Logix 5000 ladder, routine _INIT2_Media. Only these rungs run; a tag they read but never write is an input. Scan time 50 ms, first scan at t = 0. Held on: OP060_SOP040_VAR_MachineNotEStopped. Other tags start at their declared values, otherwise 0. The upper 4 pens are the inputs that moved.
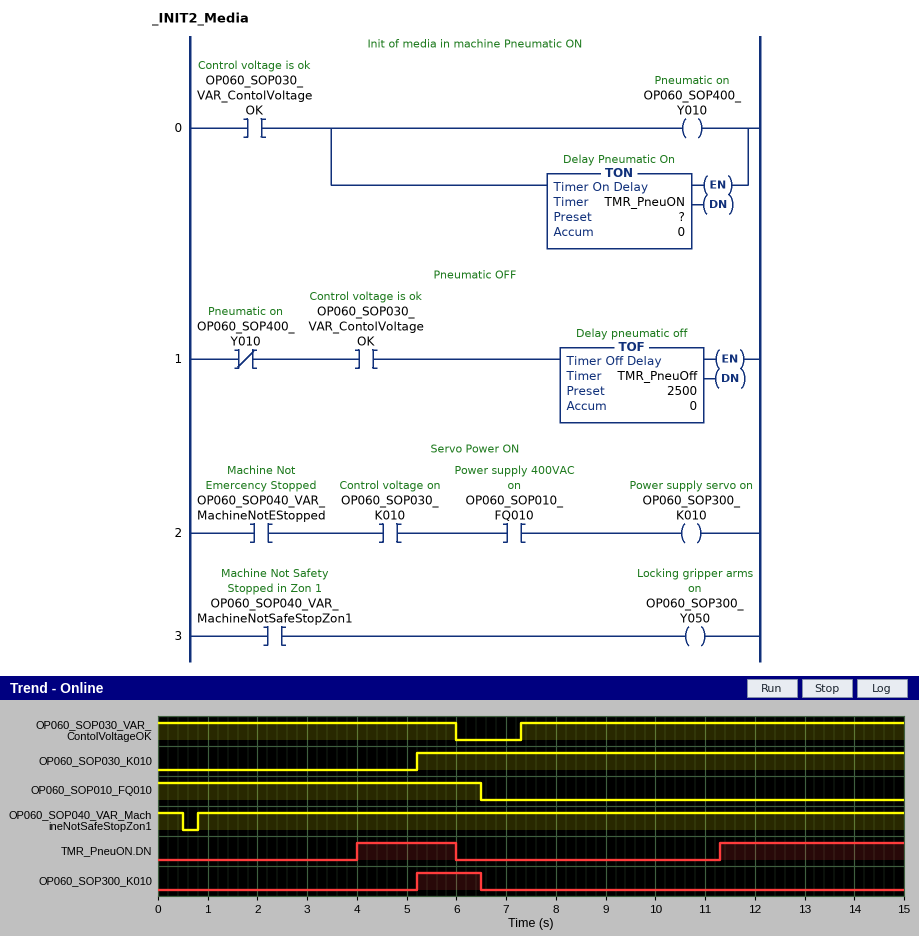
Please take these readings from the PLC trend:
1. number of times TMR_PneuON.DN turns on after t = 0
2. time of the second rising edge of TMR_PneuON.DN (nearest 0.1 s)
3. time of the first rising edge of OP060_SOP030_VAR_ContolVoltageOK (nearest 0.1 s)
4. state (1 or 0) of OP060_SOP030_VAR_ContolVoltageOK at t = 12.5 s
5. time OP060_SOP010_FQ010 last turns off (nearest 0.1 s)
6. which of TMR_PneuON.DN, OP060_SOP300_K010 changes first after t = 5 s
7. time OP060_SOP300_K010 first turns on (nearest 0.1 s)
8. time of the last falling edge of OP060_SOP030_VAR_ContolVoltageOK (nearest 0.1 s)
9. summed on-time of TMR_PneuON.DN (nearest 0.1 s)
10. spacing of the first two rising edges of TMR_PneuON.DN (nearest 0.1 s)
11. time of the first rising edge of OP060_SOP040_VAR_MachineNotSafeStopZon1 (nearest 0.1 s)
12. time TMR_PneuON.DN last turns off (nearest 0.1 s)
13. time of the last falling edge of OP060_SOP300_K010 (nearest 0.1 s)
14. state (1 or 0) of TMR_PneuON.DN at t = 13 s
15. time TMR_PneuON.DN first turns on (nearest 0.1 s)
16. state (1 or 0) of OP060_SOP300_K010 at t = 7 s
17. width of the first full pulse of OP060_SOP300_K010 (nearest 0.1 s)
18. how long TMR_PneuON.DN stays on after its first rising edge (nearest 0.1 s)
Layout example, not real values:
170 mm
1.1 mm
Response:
2
11.3 s
7.3 s
1
6.5 s
OP060_SOP300_K010
5.2 s
6.0 s
5.7 s
7.3 s
0.8 s
6.0 s
6.5 s
1
4.0 s
0
1.3 s
2.0 s
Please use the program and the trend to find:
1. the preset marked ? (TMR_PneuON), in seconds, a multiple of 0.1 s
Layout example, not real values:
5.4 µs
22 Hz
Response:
4.0 s
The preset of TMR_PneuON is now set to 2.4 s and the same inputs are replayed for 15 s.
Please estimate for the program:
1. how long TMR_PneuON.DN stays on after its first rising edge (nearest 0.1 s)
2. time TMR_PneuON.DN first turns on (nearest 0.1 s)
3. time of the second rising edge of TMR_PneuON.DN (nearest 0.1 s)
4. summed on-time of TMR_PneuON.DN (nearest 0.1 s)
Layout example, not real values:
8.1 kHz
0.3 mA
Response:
3.6 s
2.4 s
9.7 s
8.9 s
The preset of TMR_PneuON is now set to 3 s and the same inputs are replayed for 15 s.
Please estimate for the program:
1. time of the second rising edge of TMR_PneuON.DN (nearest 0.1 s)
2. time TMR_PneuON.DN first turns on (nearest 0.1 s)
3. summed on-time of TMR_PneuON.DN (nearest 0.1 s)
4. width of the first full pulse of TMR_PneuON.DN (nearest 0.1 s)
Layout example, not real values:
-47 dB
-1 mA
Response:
10.3 s
3.0 s
7.7 s
3.0 s
